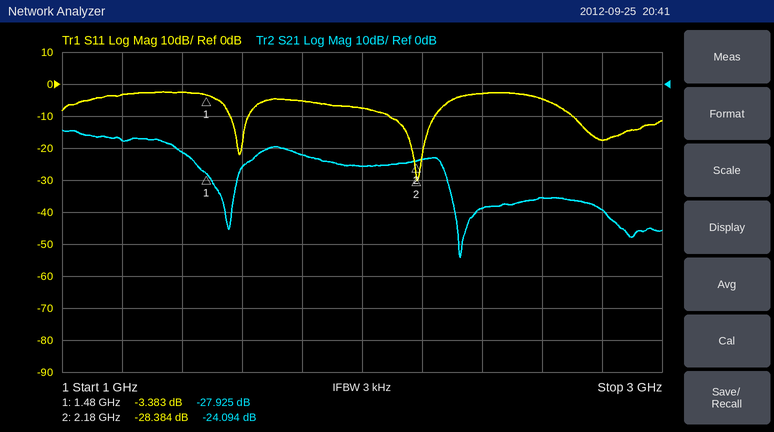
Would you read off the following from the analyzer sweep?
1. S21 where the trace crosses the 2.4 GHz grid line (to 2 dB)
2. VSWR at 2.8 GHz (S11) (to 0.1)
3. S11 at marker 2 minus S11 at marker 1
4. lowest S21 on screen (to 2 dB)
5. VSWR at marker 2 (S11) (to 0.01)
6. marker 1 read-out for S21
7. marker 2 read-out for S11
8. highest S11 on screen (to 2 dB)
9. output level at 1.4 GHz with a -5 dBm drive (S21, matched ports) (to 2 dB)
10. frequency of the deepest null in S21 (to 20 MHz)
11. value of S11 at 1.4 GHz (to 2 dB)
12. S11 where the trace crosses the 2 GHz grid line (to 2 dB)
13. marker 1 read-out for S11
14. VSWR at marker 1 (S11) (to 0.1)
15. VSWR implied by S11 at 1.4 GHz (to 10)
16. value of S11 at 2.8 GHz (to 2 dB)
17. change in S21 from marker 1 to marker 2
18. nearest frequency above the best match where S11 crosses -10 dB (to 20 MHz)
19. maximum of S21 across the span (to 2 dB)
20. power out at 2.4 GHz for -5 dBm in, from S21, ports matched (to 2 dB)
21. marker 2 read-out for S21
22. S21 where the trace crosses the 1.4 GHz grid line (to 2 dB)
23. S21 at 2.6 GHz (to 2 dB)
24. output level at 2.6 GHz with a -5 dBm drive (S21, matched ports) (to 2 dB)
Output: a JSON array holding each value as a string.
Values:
["-38 dB", "1.3", "-25.001 dB", "-54 dB", "1.08", "-27.925 dB", "-28.384 dB", "-2 dB", "-26 dBm", "2.32 GHz", "-2 dB", "-8 dB", "-3.383 dB", "5.2", "10", "-18 dB", "3.831 dB", "2.24 GHz", "-14 dB", "-44 dBm", "-24.094 dB", "-22 dB", "-36 dB", "-40 dBm"]
